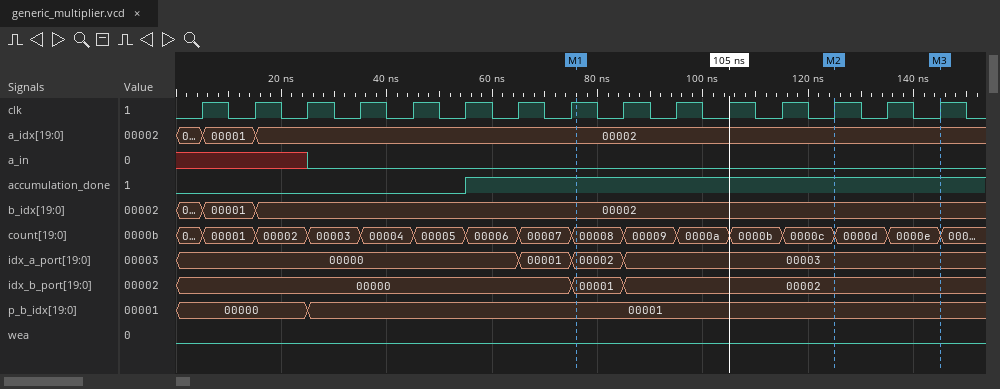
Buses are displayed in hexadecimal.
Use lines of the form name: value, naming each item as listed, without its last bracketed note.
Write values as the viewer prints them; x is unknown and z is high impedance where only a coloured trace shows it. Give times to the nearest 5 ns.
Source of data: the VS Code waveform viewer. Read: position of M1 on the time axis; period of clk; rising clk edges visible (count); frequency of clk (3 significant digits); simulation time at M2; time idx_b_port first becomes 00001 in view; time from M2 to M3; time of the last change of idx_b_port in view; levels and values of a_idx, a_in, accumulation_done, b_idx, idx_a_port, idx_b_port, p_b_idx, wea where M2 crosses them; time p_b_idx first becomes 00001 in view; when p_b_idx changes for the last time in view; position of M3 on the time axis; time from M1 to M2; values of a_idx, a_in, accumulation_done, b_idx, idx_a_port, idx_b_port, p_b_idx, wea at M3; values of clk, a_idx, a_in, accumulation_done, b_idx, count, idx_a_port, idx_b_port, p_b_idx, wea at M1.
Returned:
position of M1 on the time axis: 75 ns
period of clk: 10 ns
rising clk edges visible: 15
frequency of clk: 100 MHz
simulation time at M2: 125 ns
time idx_b_port first becomes 00001 in view: 75 ns
time from M2 to M3: 20 ns
time of the last change of idx_b_port in view: 85 ns
levels and values of a_idx, a_in, accumulation_done, b_idx, idx_a_port, idx_b_port, p_b_idx, wea where M2 crosses them: a_idx=00002, a_in=0, accumulation_done=1, b_idx=00002, idx_a_port=00003, idx_b_port=00002, p_b_idx=00001, wea=0
time p_b_idx first becomes 00001 in view: 25 ns
when p_b_idx changes for the last time in view: 25 ns
position of M3 on the time axis: 145 ns
time from M1 to M2: 50 ns
values of a_idx, a_in, accumulation_done, b_idx, idx_a_port, idx_b_port, p_b_idx, wea at M3: a_idx=00002, a_in=0, accumulation_done=1, b_idx=00002, idx_a_port=00003, idx_b_port=00002, p_b_idx=00001, wea=0
values of clk, a_idx, a_in, accumulation_done, b_idx, count, idx_a_port, idx_b_port, p_b_idx, wea at M1: clk=1, a_idx=00002, a_in=0, accumulation_done=1, b_idx=00002, count=00008, idx_a_port=00002, idx_b_port=00001, p_b_idx=00001, wea=0
